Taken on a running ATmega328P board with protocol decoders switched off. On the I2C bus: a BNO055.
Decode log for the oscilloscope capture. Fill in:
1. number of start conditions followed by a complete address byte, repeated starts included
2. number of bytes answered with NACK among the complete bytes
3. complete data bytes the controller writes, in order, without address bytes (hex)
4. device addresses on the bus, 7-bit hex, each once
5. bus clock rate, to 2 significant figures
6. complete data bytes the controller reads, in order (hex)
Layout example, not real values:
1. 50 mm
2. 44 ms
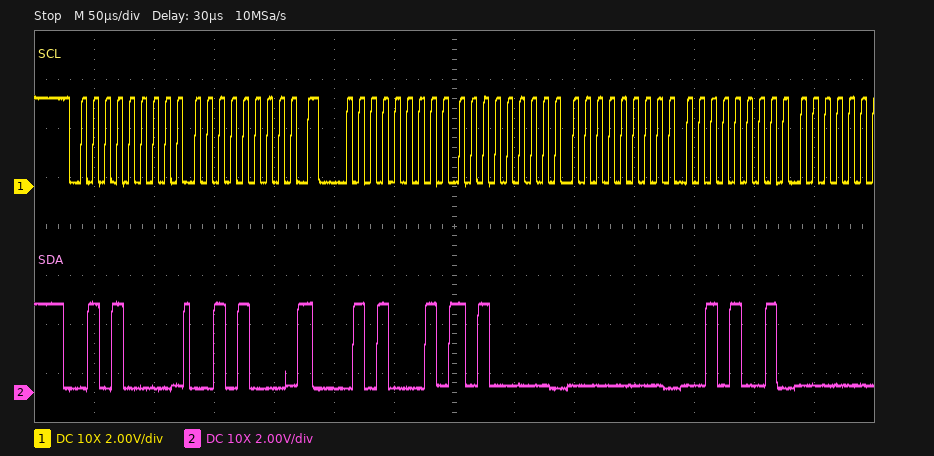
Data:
1. 2
2. 0
3. 28
4. 0x28
5. 100 kHz
6. A0 00 29
